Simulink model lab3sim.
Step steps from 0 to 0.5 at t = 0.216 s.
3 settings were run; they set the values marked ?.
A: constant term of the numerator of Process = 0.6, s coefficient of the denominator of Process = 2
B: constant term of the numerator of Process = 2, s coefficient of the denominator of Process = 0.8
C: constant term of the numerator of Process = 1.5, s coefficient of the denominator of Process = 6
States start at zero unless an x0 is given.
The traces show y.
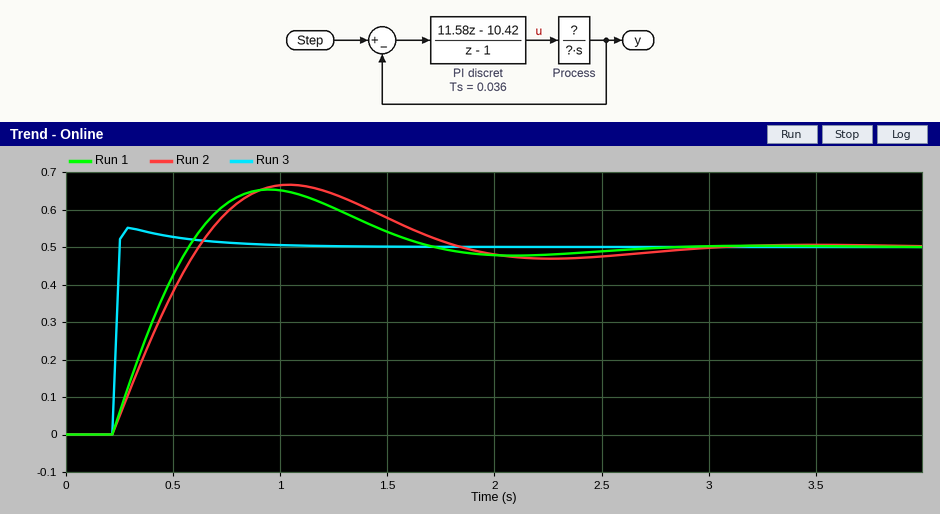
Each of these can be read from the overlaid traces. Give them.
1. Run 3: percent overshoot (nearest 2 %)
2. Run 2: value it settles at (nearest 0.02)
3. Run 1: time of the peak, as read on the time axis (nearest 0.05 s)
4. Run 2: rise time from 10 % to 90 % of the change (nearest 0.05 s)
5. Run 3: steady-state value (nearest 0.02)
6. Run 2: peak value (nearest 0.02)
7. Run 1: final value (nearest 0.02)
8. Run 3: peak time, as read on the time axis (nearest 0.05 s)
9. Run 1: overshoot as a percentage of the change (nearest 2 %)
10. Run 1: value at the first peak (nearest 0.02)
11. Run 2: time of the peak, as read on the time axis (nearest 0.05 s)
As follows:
10 %
0.50
0.95 s
0.30 s
0.50
0.66
0.50
0.30 s
30 %
0.66
1.05 s
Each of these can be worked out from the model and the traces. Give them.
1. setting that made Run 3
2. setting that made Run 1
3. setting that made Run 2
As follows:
B
A
C
